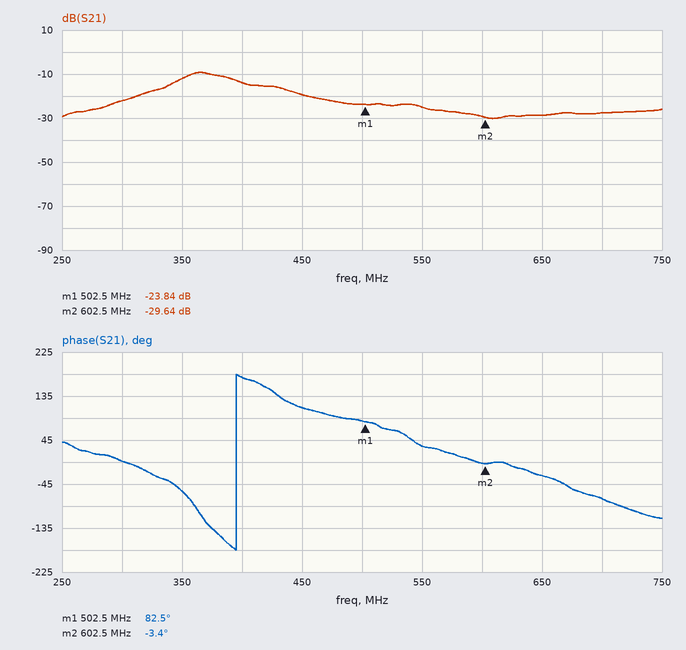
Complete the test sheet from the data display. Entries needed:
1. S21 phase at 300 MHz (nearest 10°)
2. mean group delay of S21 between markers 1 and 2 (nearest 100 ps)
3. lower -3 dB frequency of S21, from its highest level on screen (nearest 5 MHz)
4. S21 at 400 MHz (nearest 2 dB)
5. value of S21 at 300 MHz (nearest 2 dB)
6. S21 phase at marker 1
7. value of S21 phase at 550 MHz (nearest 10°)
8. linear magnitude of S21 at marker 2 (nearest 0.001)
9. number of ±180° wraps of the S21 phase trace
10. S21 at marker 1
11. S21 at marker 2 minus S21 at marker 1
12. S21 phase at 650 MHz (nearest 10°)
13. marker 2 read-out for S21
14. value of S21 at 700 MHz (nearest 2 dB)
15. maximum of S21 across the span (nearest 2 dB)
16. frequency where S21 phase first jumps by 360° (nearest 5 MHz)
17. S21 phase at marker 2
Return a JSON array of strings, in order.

["0°", "2.4 ns", "350 MHz", "-14 dB", "-22 dB", "82.5°", "30°", "0.033", "1", "-23.84 dB", "-5.80 dB", "-30°", "-29.64 dB", "-28 dB", "-10 dB", "395 MHz", "-3.4°"]
